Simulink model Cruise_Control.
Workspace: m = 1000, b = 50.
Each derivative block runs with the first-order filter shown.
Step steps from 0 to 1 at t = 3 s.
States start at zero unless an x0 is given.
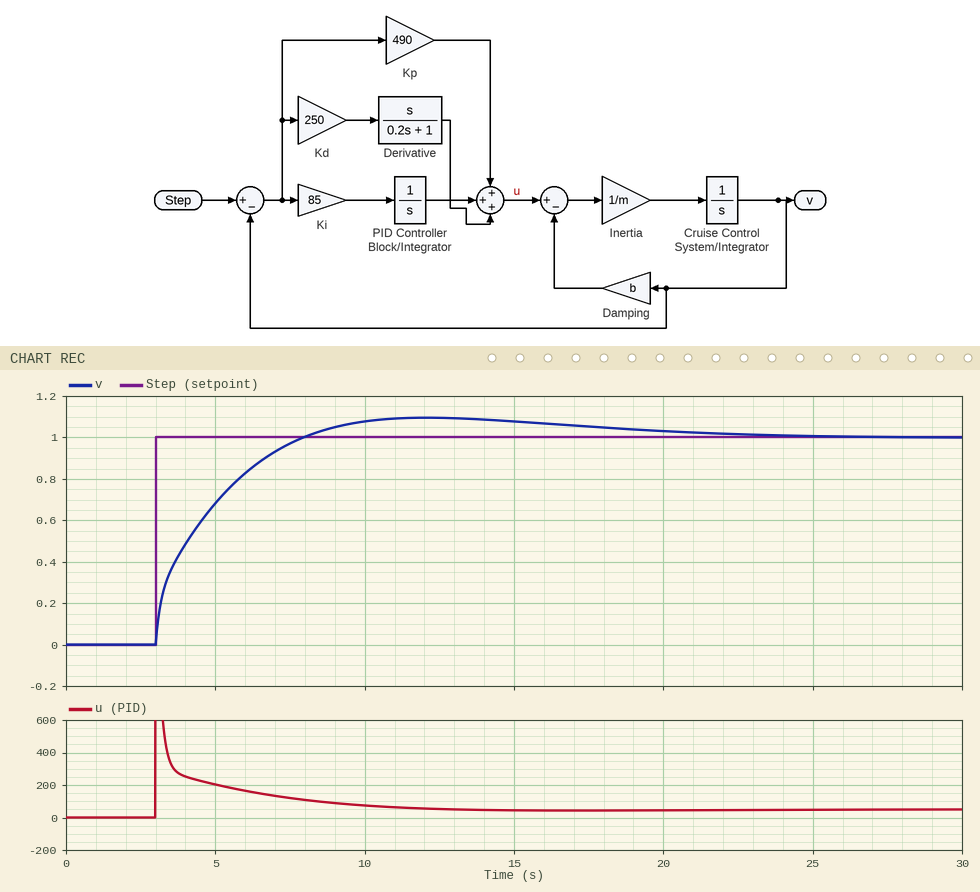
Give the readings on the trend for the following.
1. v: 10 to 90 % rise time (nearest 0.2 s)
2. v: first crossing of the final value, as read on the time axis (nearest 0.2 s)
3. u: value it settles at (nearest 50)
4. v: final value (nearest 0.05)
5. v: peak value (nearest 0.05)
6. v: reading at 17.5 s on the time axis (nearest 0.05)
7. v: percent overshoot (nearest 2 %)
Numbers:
3.6 s
8.0 s
50
1.00
1.10
1.05
10 %
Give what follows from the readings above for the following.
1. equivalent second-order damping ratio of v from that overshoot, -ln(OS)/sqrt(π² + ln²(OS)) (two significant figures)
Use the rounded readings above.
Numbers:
0.59
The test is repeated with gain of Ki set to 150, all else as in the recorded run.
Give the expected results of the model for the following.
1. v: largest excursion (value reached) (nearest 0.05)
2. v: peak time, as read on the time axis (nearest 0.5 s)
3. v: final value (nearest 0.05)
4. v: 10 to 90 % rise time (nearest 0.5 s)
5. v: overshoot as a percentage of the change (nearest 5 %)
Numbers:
1.15
10.0 s
1.00
3.0 s
15 %
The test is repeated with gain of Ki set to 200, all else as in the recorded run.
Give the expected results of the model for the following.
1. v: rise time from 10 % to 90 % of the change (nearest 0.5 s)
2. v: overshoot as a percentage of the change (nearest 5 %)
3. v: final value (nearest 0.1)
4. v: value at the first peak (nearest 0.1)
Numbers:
2.5 s
20 %
1.0
1.2
